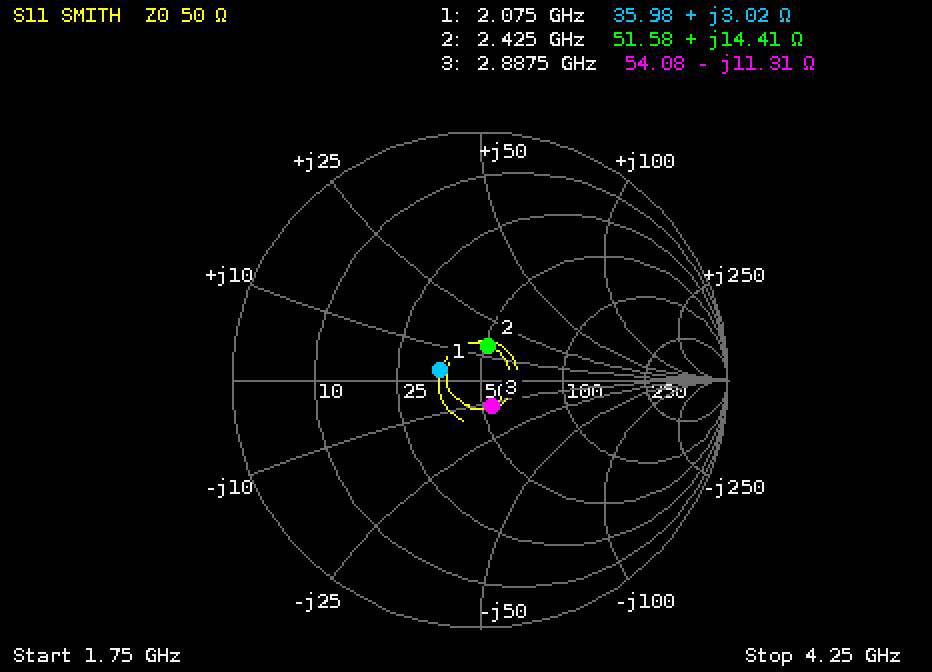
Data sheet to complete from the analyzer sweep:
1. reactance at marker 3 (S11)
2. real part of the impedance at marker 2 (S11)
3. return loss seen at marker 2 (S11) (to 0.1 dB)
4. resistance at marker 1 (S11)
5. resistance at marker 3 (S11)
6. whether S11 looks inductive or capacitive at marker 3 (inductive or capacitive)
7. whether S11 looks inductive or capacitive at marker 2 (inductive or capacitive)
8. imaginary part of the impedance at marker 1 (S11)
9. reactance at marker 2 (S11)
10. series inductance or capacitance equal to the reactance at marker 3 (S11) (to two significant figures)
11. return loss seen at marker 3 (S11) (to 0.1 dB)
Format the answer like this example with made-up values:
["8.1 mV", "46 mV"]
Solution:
["-11.31 Ω", "51.58 Ω", "17.0 dB", "35.98 Ω", "54.08 Ω", "capacitive", "inductive", "+3.02 Ω", "+14.41 Ω", "4.9 pF", "18.8 dB"]
